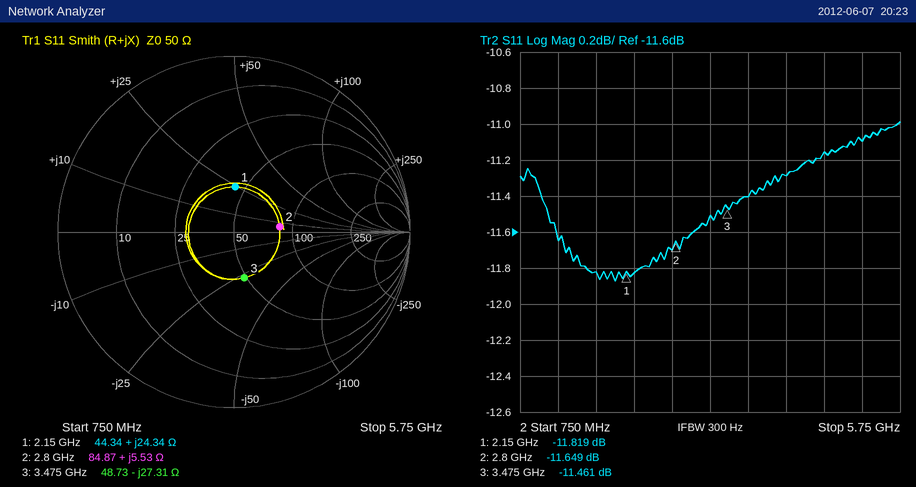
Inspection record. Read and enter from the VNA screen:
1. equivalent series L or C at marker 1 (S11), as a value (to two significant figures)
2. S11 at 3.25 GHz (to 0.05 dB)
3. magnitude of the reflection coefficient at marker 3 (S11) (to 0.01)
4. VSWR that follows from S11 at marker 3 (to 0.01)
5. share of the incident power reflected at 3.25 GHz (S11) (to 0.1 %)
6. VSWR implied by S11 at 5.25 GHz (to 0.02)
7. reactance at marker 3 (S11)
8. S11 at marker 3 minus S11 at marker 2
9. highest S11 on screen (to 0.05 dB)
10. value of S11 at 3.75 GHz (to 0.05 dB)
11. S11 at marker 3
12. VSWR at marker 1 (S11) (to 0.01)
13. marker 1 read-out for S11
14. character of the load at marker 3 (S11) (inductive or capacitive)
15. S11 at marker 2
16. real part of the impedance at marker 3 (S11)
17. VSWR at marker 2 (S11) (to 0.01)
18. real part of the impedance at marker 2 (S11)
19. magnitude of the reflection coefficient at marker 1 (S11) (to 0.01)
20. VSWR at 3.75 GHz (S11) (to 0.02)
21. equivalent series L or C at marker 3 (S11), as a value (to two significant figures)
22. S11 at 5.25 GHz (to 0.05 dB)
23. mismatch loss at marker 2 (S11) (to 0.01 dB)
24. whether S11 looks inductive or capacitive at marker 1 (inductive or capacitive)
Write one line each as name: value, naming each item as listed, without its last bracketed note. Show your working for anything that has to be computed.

equivalent series L or C at marker 1 (S11), as a value: L = 24.34 Ω/(2π × 2.15 GHz) ≈ 1.8 nH
S11 at 3.25 GHz: -11.50 dB
magnitude of the reflection coefficient at marker 3 (S11): 0.27
VSWR that follows from S11 at marker 3: (1 + 0.2673)/(1 − 0.2673) ≈ 1.73
share of the incident power reflected at 3.25 GHz (S11): 10^(-11.5/10) ≈ 7.1 %
VSWR implied by S11 at 5.25 GHz: |Γ| = 10^(-11.1/20) = 0.2786; VSWR = (1 + 0.2786)/(1 − 0.2786) ≈ 1.77, so 1.78 to the nearest 0.02
reactance at marker 3: -27.31 Ω
S11 at marker 3 minus S11 at marker 2: -11.461 − (-11.649) = 0.188 dB
highest S11 on screen: -11.00 dB
value of S11 at 3.75 GHz: -11.40 dB
S11 at marker 3: -11.461 dB
VSWR at marker 1 (S11): 1.69
marker 1 read-out for S11: -11.819 dB
character of the load at marker 3 (S11): capacitive
S11 at marker 2: -11.649 dB
real part of the impedance at marker 3: 48.73 Ω
VSWR at marker 2 (S11): 1.71
real part of the impedance at marker 2: 84.87 Ω
magnitude of the reflection coefficient at marker 1 (S11): 10^(-11.819/20) ≈ 0.26
VSWR at 3.75 GHz (S11): |Γ| = 10^(-11.4/20) = 0.2692; VSWR = (1 + 0.2692)/(1 − 0.2692) ≈ 1.74
equivalent series L or C at marker 3 (S11), as a value: C = 1/(2π × 3.475 GHz × 27.31 Ω) ≈ 1.7 pF
S11 at 5.25 GHz: -11.10 dB
mismatch loss at marker 2 (S11): −10 log10(1 − 10^(-11.649/10)) ≈ 0.31 dB
whether S11 looks inductive or capacitive at marker 1: inductive
